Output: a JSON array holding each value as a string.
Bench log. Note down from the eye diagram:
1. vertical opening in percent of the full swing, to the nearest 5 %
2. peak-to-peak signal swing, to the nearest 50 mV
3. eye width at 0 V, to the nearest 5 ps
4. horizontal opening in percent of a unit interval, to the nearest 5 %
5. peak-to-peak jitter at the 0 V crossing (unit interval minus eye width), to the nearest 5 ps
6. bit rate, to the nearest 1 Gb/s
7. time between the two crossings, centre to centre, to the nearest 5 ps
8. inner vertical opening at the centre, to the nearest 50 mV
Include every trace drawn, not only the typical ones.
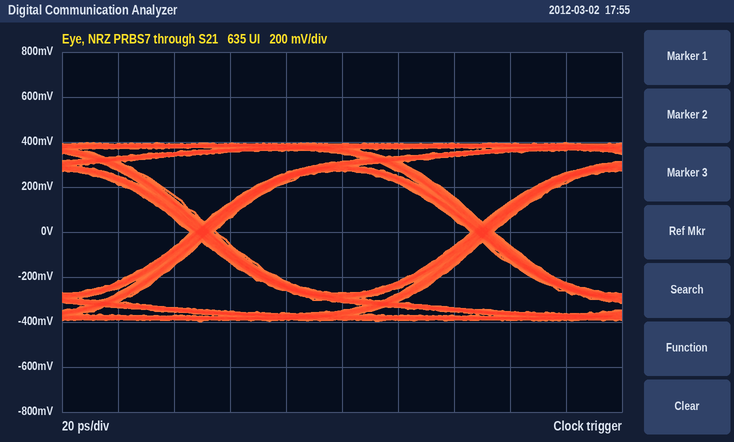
["70 %", "800 mV", "90 ps", "90 %", "10 ps", "10 Gb/s", "100 ps", "550 mV"]
